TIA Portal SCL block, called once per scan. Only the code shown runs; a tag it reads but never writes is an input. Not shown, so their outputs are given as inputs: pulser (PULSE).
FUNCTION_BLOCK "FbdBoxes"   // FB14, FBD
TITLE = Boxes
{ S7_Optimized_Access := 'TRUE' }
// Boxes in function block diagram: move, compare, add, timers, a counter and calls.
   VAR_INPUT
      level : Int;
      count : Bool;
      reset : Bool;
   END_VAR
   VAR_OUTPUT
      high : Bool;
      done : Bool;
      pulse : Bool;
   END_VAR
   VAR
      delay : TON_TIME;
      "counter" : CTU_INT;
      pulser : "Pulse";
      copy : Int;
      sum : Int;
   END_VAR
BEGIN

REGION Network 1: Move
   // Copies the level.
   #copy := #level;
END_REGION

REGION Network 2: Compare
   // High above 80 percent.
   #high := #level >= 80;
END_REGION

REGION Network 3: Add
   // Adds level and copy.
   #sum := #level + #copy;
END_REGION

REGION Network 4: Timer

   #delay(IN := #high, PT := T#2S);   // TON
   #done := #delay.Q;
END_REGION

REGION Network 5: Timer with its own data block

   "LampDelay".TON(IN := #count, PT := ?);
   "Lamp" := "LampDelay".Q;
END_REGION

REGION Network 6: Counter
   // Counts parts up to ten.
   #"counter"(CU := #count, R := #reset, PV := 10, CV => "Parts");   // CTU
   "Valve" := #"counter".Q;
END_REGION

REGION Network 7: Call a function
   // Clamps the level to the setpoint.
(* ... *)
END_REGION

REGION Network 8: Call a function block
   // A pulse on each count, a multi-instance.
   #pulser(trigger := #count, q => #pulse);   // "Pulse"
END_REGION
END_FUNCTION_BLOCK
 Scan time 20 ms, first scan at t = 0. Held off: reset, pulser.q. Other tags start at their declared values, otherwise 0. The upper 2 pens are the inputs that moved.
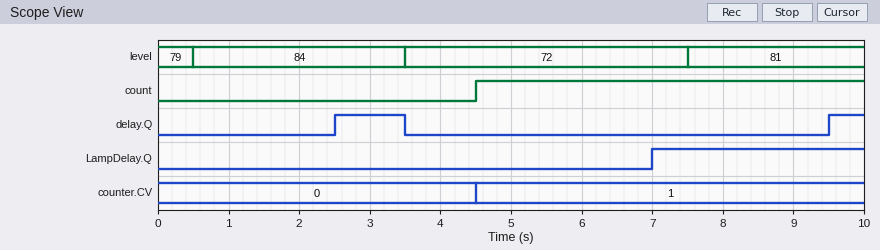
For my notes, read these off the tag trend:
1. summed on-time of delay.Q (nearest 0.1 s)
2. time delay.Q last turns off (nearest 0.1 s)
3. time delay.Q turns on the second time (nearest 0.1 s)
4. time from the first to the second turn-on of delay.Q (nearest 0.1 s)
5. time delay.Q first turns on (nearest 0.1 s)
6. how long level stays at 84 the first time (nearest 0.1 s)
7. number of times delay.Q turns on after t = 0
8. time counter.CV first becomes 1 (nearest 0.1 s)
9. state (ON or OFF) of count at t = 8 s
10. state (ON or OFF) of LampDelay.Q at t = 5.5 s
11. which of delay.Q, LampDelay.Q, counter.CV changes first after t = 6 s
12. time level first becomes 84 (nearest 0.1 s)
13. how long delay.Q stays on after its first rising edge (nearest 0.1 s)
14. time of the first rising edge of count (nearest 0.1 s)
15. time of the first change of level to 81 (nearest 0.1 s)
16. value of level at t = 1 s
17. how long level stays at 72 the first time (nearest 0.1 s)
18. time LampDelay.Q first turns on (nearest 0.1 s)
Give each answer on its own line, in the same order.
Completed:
1.5 s
3.5 s
9.5 s
7.0 s
2.5 s
3.0 s
2
4.5 s
ON
OFF
LampDelay.Q
0.5 s
1.0 s
4.5 s
7.5 s
84
4.0 s
7.0 s
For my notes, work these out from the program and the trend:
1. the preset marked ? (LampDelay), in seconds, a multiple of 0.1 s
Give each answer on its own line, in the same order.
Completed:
2.5 s
